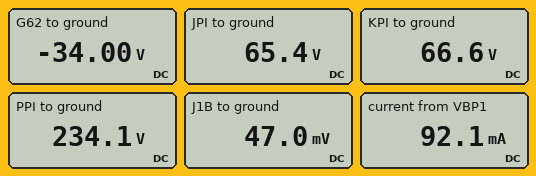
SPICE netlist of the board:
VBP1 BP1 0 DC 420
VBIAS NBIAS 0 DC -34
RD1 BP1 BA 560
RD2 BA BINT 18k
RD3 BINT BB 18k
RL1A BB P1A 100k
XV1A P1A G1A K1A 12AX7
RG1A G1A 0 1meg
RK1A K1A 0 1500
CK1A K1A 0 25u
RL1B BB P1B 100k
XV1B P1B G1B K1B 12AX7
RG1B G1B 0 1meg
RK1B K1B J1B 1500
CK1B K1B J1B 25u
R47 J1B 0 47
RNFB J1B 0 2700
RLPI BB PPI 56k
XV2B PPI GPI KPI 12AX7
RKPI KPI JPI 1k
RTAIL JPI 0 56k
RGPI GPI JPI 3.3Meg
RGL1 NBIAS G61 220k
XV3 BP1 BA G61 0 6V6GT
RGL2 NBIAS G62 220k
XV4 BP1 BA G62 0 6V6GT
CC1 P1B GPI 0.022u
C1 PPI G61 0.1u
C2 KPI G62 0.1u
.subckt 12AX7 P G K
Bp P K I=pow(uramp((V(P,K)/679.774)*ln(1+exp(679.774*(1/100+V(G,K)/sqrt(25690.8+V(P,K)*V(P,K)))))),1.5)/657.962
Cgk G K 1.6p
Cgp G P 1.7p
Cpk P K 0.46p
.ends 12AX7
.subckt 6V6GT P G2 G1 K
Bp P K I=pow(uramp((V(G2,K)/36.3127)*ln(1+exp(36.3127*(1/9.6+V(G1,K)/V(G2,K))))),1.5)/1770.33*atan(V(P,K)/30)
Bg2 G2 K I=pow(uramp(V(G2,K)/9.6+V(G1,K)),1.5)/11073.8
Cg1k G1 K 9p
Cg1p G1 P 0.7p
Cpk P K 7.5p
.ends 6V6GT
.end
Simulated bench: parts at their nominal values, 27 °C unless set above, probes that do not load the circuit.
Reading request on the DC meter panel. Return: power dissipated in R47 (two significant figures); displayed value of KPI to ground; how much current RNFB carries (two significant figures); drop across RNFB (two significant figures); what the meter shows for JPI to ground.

47 µW
66.6 V
17 µA
47 mV
65.4 V
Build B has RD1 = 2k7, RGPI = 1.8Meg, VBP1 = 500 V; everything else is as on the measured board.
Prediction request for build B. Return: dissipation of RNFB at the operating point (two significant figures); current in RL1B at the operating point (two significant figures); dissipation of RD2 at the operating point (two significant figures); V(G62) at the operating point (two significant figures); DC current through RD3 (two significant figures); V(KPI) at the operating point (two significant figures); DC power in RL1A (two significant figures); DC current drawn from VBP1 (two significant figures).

1.0 µW
1.1 mA
230 mW
-34 V
3.6 mA
74 V
130 mW
140 mA
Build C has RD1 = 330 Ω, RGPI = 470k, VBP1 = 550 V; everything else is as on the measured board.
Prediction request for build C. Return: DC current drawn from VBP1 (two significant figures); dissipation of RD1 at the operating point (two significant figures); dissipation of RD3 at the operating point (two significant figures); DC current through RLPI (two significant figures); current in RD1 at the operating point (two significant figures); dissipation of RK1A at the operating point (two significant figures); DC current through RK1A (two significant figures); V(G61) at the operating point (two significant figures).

240 mA
180 mW
310 mW
1.5 mA
23 mA
2.7 mW
1.3 mA
-34 V
